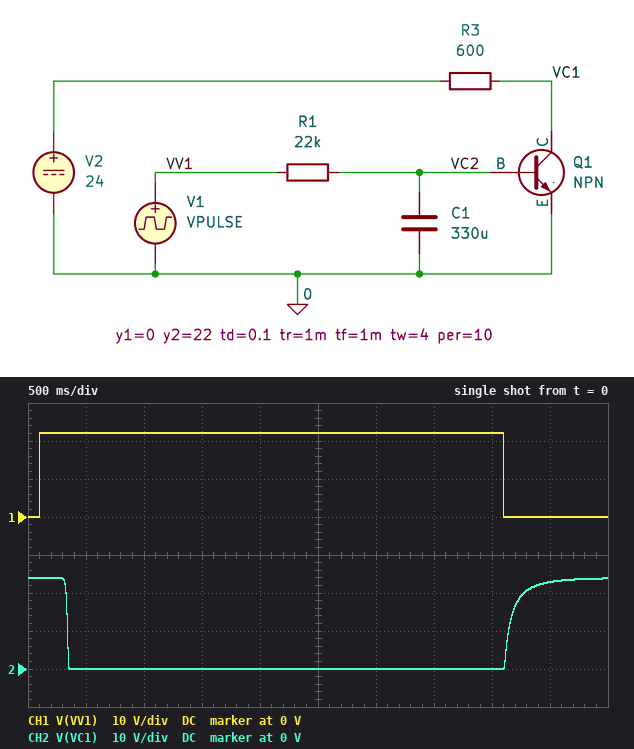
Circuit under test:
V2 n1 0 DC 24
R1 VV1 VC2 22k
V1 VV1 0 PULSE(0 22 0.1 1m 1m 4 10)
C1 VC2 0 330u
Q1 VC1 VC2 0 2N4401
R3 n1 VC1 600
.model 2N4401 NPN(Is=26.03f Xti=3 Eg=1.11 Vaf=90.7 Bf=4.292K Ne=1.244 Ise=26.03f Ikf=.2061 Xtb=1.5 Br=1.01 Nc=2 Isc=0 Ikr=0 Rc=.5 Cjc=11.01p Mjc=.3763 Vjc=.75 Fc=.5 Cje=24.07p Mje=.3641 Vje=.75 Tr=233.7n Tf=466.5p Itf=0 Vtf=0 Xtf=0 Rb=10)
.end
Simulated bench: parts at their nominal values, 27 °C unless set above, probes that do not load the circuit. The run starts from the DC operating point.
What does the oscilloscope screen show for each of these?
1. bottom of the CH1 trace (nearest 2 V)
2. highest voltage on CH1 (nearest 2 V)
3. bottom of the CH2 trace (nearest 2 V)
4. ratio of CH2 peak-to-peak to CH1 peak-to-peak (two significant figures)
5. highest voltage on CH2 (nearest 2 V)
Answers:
0 V
22 V
0 V
1.1
24 V
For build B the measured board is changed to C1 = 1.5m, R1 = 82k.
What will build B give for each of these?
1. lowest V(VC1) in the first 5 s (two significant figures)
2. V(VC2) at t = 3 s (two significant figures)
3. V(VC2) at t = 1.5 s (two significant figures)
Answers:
16 V
510 mV
250 mV
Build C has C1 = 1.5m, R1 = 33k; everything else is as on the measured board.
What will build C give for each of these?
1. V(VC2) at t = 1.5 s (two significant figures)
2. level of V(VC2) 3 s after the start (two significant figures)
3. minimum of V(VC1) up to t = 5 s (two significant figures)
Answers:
610 mV
740 mV
140 mV
